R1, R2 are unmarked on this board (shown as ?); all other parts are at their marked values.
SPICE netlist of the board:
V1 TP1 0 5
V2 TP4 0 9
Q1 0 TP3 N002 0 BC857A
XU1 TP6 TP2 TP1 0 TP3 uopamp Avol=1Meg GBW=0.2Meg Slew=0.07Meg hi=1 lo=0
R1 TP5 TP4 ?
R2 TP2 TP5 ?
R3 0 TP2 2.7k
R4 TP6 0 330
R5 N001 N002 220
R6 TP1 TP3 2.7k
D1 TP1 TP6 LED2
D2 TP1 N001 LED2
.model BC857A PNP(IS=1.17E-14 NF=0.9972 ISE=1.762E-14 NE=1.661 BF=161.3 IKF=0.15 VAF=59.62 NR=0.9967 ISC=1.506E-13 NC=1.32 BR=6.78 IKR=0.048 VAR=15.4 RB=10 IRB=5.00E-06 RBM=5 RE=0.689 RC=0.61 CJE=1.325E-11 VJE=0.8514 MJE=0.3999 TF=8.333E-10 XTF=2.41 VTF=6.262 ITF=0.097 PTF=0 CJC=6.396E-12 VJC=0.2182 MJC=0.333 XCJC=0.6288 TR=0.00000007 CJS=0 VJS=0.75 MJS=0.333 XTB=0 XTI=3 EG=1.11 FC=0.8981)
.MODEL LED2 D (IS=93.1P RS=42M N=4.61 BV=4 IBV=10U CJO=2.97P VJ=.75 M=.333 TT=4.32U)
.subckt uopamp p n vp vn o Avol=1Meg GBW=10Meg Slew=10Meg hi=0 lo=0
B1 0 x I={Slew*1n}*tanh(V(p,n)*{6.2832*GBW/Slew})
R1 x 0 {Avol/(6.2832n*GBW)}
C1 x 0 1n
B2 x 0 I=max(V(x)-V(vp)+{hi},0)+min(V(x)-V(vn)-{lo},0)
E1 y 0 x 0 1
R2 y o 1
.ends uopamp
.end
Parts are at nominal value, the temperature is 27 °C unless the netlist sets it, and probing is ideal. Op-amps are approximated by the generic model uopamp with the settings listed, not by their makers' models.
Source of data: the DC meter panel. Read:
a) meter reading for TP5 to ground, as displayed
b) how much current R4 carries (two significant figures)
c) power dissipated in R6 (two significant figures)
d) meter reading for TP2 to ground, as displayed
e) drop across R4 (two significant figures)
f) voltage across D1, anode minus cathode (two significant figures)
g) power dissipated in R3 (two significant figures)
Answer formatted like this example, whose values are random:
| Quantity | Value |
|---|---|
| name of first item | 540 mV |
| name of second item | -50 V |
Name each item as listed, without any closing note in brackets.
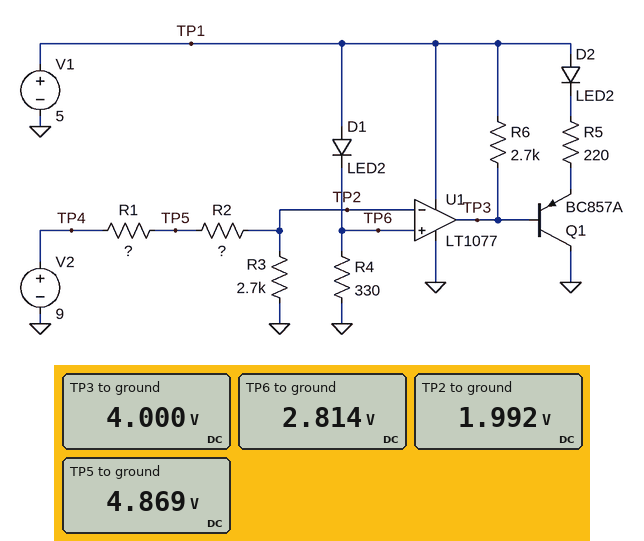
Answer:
| Quantity | Value |
|---|---|
| meter reading for TP5 to ground, as displayed | 4.869 V |
| how much current R4 carries | 8.5 mA |
| power dissipated in R6 | 370 µW |
| meter reading for TP2 to ground, as displayed | 1.992 V |
| drop across R4 | 2.8 V |
| voltage across D1, anode minus cathode | 2.2 V |
| power dissipated in R3 | 1.5 mW |
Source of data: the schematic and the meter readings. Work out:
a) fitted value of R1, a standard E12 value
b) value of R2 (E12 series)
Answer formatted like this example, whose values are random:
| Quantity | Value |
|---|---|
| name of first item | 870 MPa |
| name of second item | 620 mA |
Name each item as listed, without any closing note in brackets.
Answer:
| Quantity | Value |
|---|---|
| fitted value of R1, a standard E12 value | 5.6 kΩ |
| value of R2 | 3.9 kΩ |
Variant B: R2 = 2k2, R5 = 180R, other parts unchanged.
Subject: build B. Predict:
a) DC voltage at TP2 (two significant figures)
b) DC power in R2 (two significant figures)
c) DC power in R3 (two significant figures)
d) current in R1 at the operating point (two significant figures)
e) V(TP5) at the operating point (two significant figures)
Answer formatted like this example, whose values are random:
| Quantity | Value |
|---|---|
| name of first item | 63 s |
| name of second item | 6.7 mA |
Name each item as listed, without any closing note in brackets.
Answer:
| Quantity | Value |
|---|---|
| DC voltage at TP2 | 2.3 V |
| DC power in R2 | 1.6 mW |
| DC power in R3 | 2.0 mW |
| current in R1 at the operating point | 860 µA |
| V(TP5) at the operating point | 4.2 V |
